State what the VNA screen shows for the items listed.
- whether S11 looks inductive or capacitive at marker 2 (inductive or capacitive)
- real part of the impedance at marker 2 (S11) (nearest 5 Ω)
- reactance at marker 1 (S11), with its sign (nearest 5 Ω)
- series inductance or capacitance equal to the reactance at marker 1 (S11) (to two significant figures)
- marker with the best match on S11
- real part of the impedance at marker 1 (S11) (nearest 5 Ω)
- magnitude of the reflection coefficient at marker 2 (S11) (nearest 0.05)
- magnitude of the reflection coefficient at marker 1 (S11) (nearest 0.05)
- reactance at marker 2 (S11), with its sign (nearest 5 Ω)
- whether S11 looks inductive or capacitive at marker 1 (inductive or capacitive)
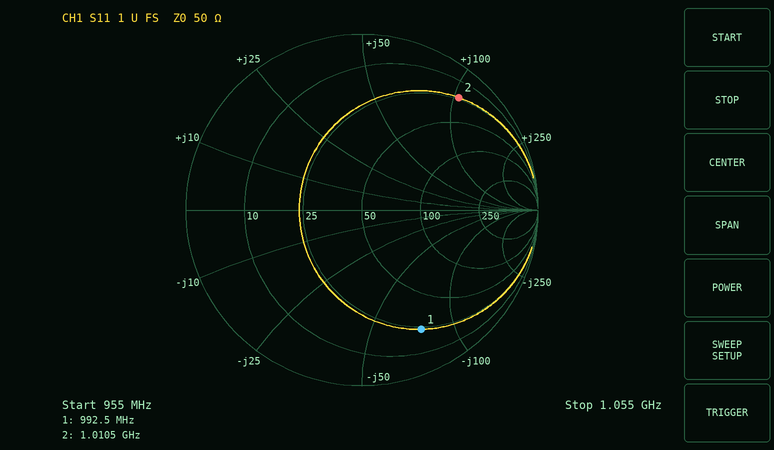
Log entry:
inductive
25 Ω
-75 Ω
2.1 pF
marker 1
25 Ω
0.85
0.75
+105 Ω
capacitive
